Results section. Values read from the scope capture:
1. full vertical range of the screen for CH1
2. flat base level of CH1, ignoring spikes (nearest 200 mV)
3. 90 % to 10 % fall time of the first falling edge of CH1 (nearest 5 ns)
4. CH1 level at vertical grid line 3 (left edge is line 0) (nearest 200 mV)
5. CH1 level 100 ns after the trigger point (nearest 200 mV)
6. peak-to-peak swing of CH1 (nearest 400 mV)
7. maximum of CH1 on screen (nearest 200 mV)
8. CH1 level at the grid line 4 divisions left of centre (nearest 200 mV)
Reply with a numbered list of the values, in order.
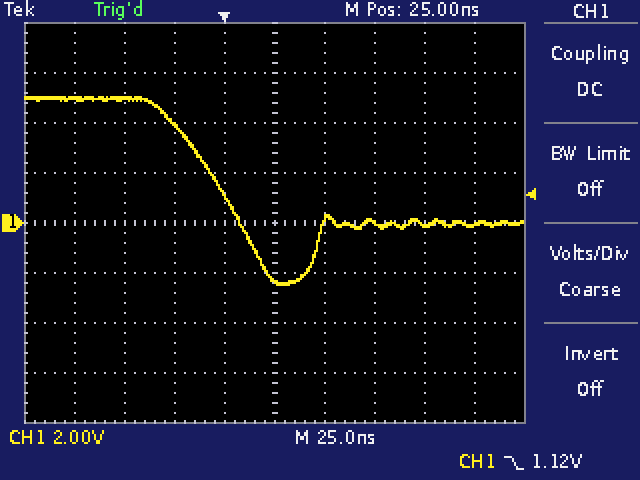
1. 16 V
2. 0.0 V
3. 35 ns
4. 4.0 V
5. 0.0 V
6. 7.6 V
7. 5.0 V
8. 5.0 V
